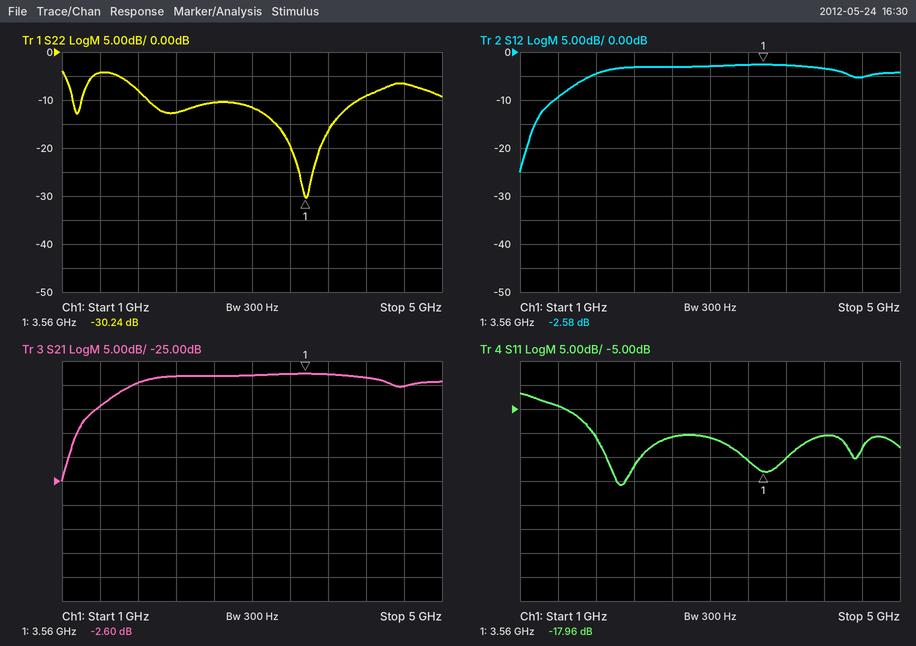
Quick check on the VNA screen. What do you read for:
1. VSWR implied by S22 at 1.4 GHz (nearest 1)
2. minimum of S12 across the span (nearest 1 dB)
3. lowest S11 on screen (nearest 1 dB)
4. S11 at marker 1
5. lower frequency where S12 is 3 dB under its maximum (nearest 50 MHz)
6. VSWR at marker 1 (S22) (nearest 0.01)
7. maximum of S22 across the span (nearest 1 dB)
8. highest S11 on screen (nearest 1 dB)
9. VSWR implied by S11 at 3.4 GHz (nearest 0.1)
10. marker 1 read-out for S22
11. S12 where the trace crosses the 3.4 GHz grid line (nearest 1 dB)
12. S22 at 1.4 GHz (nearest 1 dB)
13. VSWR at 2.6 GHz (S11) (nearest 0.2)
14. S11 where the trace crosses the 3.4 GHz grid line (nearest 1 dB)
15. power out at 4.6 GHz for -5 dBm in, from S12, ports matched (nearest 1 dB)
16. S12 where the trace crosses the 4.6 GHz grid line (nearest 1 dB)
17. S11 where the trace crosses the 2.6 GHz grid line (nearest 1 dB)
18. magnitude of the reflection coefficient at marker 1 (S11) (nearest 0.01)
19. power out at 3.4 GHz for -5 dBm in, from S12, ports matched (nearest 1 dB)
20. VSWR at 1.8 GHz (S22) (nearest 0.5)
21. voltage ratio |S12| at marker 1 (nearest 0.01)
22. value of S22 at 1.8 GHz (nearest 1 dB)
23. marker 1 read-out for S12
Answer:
4
-25 dB
-21 dB
-17.96 dB
1.70 GHz
1.06
-4 dB
-2 dB
1.4
-30.24 dB
-3 dB
-4 dB
1.8
-16 dB
-10 dBm
-5 dB
-11 dB
0.13
-8 dBm
2.5
0.74
-8 dB
-2.58 dB
